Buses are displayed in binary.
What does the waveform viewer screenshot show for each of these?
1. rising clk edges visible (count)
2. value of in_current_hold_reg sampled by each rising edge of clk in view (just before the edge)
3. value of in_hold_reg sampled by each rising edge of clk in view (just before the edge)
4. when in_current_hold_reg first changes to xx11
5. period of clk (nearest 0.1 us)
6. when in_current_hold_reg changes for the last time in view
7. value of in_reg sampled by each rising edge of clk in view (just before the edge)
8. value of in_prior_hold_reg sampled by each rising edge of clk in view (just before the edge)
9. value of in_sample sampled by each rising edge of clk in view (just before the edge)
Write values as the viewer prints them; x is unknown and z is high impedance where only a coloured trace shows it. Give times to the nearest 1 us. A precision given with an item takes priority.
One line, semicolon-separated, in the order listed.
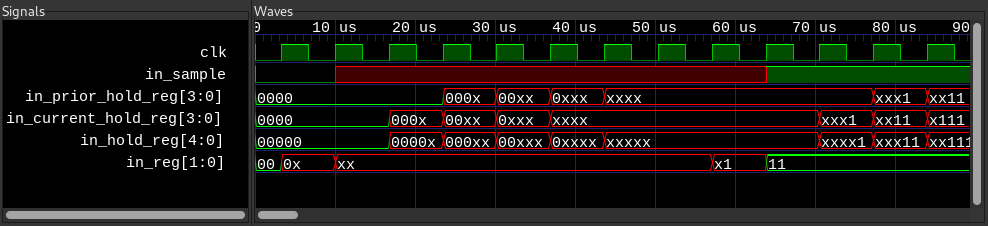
13; 0000, 0000, 0000, 000x, 00xx, 0xxx, xxxx, xxxx, xxxx, xxxx, xxxx, xxx1, xx11; 00000, 00000, 00000, 0000x, 000xx, 00xxx, 0xxxx, xxxxx, xxxxx, xxxxx, xxxxx, xxxx1, xxx11; 77 us; 6.7 us; 84 us; 00, 0x, xx, xx, xx, xx, xx, xx, xx, x1, 11, 11, 11; 0000, 0000, 0000, 0000, 000x, 00xx, 0xxx, xxxx, xxxx, xxxx, xxxx, xxxx, xxx1; 0 0 x x x x x x x x 1 1 1
